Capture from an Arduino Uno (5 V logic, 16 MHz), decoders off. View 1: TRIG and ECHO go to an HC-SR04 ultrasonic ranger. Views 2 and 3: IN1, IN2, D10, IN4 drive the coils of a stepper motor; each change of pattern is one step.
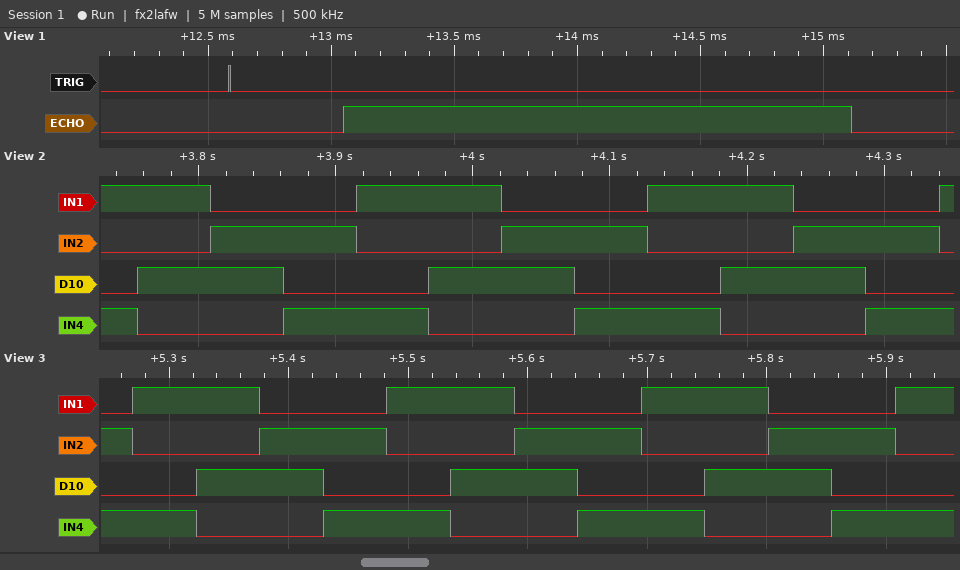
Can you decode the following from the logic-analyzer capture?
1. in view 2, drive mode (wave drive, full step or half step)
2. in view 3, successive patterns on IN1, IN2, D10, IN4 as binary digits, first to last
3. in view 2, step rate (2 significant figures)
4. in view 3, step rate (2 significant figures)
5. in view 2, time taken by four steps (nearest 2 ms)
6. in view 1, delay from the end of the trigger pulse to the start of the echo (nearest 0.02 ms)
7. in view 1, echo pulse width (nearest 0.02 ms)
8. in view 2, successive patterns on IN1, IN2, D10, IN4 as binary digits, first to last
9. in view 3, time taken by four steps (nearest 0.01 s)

full step
0101 1001 1010 0110 0101 1001 1010 0110 0101 1001 1010 0110 0101 1001
19 steps/s
19 steps/s
212 ms
0.46 ms
2.06 ms
1001 1010 0110 0101 1001 1010 0110 0101 1001 1010 0110 0101 1001
0.21 s
